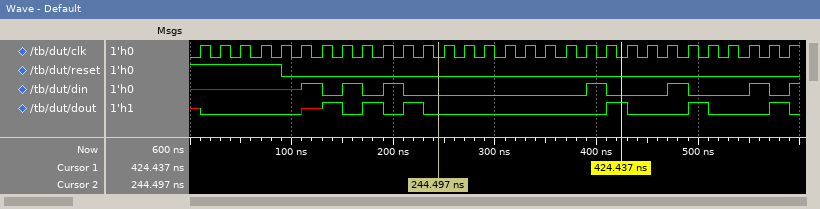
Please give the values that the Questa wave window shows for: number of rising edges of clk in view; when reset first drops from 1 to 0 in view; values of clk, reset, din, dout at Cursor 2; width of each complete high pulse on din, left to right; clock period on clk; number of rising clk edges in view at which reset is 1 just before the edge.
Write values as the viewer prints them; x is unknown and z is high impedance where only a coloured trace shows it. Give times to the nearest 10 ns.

30
90 ns
clk=0, reset=0, din=0, dout=0
20 ns, 20 ns, 20 ns, 20 ns, 20 ns
20 ns
5
